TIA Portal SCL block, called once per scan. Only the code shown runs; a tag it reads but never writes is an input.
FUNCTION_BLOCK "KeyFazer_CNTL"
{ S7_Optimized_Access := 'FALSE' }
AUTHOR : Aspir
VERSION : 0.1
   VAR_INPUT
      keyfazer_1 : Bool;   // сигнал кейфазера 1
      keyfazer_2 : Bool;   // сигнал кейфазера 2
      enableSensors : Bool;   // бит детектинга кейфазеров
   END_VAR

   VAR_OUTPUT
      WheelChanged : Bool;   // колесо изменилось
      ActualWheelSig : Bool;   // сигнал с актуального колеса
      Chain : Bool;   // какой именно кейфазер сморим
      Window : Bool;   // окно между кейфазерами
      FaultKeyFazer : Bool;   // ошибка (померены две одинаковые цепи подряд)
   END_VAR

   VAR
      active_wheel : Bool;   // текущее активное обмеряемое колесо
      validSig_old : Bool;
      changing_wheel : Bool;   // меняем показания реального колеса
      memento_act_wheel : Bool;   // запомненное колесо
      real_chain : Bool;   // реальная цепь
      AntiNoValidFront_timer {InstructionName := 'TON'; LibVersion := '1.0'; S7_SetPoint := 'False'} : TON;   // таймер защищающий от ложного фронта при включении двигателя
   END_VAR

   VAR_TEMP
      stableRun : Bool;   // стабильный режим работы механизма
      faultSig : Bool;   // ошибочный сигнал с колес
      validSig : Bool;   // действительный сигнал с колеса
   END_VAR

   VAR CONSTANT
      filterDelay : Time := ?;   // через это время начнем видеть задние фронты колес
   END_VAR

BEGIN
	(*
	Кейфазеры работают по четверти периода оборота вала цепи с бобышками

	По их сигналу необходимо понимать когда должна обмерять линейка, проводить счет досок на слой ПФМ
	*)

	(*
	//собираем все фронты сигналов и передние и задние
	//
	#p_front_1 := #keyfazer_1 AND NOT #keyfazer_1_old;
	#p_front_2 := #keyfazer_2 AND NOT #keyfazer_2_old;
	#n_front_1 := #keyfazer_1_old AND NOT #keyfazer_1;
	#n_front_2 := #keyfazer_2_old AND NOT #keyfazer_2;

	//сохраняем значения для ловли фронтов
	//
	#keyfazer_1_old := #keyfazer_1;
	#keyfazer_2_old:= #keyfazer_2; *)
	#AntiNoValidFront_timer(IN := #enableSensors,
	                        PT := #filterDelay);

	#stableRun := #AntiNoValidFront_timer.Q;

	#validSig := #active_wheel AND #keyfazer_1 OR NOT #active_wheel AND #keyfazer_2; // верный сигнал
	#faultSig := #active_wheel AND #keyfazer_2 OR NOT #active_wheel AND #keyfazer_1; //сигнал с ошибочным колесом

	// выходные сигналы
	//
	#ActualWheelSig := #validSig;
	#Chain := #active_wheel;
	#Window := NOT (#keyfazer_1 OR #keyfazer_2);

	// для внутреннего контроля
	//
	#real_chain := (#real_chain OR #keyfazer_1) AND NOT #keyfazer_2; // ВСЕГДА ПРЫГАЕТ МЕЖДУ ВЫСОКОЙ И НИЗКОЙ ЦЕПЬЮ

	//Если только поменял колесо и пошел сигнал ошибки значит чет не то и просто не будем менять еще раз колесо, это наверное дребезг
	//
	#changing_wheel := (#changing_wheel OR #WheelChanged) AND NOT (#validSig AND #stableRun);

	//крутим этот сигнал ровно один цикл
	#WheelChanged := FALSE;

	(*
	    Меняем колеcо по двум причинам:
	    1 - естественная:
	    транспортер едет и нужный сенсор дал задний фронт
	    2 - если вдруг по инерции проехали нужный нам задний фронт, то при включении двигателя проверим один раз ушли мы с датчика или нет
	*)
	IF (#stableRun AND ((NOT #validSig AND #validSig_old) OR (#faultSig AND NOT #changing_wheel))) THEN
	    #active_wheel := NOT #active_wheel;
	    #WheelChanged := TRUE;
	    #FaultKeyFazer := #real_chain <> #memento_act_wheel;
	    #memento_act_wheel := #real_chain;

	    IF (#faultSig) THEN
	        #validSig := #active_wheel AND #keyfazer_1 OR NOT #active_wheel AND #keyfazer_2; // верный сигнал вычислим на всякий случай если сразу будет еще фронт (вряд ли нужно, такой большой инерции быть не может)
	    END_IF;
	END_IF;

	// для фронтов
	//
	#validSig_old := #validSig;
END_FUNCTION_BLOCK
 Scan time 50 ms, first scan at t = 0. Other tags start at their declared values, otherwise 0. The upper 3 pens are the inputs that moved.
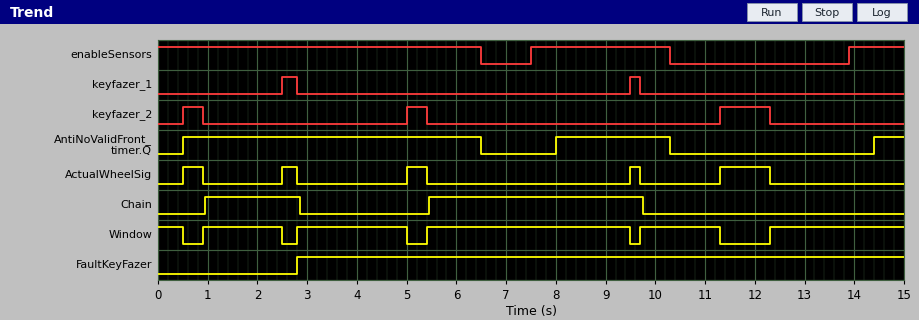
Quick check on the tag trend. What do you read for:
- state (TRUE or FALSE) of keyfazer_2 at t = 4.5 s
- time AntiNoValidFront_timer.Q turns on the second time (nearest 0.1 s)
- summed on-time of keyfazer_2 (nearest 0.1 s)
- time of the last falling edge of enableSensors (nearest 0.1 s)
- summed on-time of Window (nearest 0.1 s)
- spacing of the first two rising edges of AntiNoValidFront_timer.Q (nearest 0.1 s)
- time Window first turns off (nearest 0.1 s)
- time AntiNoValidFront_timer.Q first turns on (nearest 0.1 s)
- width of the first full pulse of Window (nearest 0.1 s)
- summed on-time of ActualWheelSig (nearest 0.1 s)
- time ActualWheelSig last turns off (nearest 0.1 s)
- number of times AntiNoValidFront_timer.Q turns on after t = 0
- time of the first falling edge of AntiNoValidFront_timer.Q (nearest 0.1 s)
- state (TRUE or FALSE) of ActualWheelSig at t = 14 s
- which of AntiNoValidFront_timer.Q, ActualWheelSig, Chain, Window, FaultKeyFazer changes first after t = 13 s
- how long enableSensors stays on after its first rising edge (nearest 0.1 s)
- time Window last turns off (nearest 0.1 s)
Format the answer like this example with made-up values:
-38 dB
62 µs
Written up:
FALSE
8.0 s
1.8 s
10.3 s
12.7 s
7.5 s
0.5 s
0.5 s
1.6 s
2.3 s
12.3 s
3
6.5 s
FALSE
AntiNoValidFront_timer.Q
2.8 s
11.3 s
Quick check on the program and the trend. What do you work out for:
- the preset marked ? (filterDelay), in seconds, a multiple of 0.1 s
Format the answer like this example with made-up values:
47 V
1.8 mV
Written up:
0.5 s
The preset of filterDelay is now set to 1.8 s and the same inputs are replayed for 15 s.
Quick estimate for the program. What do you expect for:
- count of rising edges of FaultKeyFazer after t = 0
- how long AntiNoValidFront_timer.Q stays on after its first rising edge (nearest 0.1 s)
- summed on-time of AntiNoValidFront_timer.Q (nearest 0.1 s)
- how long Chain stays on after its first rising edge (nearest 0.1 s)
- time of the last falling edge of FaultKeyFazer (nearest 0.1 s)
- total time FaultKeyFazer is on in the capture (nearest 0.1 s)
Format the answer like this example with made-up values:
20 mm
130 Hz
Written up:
2
4.7 s
5.7 s
0.3 s
2.8 s
9.9 s
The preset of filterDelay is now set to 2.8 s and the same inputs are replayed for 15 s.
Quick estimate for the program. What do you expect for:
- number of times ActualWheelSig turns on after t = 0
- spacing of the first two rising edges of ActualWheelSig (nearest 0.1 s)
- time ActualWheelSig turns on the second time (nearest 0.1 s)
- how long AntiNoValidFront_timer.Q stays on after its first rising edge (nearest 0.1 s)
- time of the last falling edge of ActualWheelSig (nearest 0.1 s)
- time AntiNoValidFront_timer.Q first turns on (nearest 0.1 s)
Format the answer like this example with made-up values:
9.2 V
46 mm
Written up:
3
4.5 s
5.0 s
3.7 s
9.7 s
2.8 s
